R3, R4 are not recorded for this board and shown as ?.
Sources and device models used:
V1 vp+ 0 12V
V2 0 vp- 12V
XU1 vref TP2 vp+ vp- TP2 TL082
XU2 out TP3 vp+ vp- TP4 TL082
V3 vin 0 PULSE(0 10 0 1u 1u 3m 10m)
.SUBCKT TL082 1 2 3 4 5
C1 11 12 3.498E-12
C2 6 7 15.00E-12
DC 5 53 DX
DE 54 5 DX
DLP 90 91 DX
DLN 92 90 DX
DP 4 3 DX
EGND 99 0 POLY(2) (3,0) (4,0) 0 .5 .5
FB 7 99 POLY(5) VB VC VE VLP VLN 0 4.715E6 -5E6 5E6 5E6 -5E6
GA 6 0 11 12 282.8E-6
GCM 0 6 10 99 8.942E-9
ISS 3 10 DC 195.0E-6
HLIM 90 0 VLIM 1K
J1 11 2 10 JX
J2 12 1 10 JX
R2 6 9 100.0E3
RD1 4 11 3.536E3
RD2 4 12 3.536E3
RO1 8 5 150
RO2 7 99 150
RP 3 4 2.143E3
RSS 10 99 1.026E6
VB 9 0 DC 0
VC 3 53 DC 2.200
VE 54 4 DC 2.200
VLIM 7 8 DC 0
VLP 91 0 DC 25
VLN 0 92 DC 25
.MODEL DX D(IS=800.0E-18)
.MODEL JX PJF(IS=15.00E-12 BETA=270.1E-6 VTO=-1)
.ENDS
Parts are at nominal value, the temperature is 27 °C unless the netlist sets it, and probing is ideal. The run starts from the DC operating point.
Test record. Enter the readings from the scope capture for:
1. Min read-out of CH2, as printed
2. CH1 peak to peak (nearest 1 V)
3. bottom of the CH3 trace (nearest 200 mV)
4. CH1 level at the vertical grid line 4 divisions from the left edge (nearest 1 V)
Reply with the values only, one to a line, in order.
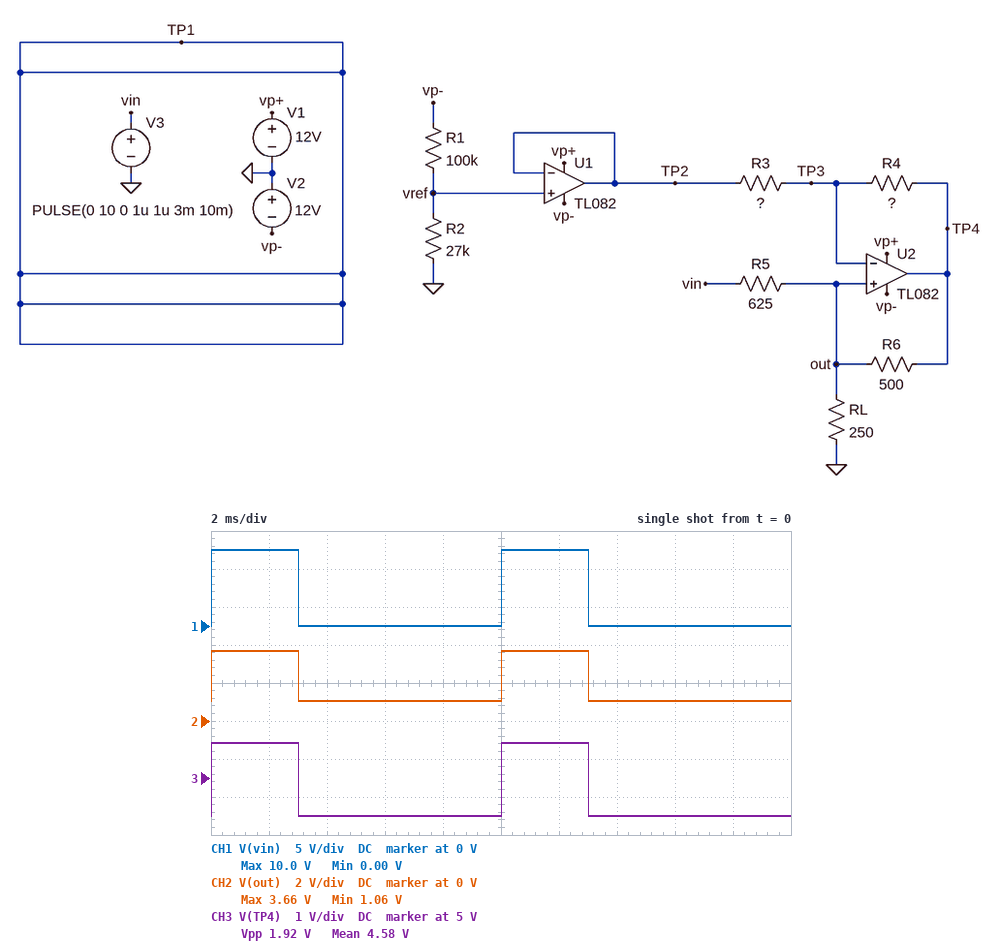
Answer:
1.06 V
10 V
4.0 V
0 V
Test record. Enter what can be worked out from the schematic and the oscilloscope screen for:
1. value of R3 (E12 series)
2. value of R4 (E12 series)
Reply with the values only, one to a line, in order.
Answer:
220 Ω
180 Ω
